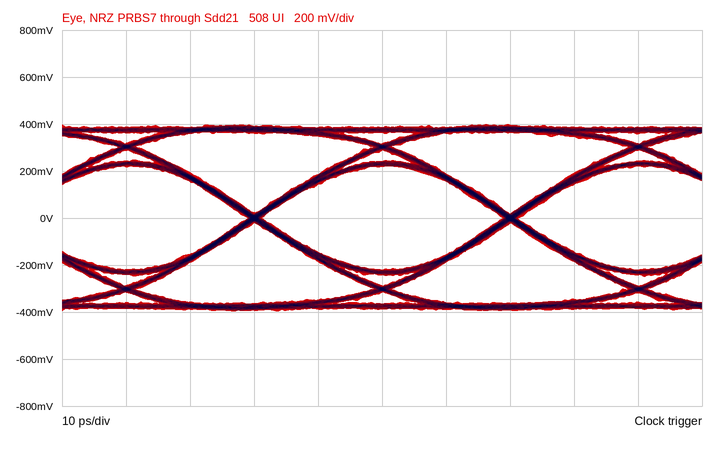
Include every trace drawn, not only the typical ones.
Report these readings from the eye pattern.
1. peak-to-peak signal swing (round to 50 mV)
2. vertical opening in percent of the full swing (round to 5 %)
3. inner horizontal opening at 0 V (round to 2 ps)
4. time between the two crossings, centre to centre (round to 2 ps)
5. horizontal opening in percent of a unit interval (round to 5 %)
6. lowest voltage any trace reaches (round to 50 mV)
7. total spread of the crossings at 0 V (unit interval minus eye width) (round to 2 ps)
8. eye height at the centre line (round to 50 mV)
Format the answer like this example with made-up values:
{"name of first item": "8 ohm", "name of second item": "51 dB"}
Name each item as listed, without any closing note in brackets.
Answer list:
{"peak-to-peak signal swing": "800 mV", "vertical opening in percent of the full swing": "55 %", "inner horizontal opening at 0 V": "38 ps", "time between the two crossings, centre to centre": "40 ps", "horizontal opening in percent of a unit interval": "95 %", "lowest voltage any trace reaches": "-400 mV", "total spread of the crossings at 0 V (unit interval minus eye width)": "2 ps", "eye height at the centre line": "450 mV"}
